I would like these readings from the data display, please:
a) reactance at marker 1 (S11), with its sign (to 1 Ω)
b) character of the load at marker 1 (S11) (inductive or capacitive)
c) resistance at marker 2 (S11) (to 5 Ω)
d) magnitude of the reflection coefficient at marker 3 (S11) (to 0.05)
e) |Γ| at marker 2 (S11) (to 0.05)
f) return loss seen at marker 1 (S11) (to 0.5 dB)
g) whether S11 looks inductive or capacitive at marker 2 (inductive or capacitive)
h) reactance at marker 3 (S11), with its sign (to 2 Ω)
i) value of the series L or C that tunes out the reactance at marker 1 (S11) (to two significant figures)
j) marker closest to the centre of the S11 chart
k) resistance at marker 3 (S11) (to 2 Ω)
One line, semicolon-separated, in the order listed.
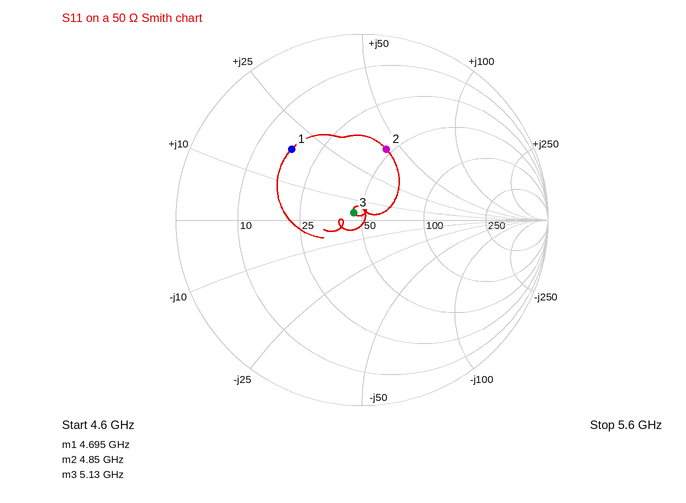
+19 Ω; inductive; 45 Ω; 0.05; 0.40; 5.5 dB; inductive; +4 Ω; 1.8 pF; marker 3; 46 Ω
